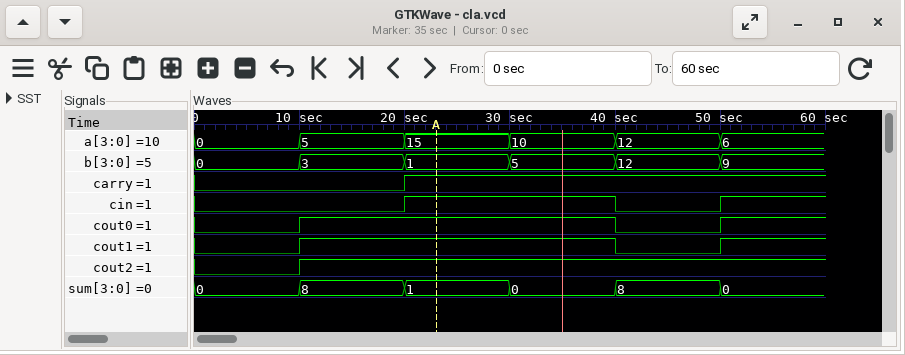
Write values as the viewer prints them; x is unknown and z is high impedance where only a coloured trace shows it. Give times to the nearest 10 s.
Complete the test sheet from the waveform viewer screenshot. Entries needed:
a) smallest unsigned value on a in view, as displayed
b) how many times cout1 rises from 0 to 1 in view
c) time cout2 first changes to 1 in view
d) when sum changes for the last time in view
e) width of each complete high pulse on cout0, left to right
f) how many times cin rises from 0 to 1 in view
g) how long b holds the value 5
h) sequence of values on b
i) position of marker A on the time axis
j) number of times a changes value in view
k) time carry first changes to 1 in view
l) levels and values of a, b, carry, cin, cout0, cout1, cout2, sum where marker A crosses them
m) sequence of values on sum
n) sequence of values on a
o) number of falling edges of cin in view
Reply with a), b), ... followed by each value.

a) 0
b) 2
c) 10 s
d) 50 s
e) 30 s
f) 2
g) 10 s
h) 0, 3, 1, 5, 12, 9
i) 20 s
j) 5
k) 20 s
l) a=15, b=1, carry=1, cin=1, cout0=1, cout1=1, cout2=1, sum=1
m) 0, 8, 1, 0, 8, 0
n) 0, 5, 15, 10, 12, 6
o) 1
